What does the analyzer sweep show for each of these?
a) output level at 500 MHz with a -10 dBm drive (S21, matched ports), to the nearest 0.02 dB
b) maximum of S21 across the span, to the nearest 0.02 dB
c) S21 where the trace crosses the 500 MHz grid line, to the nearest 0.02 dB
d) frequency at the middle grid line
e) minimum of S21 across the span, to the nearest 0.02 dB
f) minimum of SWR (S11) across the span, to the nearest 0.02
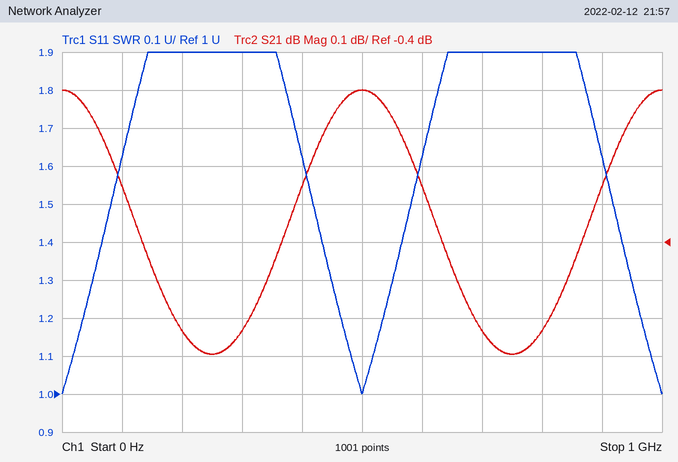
-10.00 dBm
0.00 dB
0.00 dB
500 MHz
-0.70 dB
1.00
